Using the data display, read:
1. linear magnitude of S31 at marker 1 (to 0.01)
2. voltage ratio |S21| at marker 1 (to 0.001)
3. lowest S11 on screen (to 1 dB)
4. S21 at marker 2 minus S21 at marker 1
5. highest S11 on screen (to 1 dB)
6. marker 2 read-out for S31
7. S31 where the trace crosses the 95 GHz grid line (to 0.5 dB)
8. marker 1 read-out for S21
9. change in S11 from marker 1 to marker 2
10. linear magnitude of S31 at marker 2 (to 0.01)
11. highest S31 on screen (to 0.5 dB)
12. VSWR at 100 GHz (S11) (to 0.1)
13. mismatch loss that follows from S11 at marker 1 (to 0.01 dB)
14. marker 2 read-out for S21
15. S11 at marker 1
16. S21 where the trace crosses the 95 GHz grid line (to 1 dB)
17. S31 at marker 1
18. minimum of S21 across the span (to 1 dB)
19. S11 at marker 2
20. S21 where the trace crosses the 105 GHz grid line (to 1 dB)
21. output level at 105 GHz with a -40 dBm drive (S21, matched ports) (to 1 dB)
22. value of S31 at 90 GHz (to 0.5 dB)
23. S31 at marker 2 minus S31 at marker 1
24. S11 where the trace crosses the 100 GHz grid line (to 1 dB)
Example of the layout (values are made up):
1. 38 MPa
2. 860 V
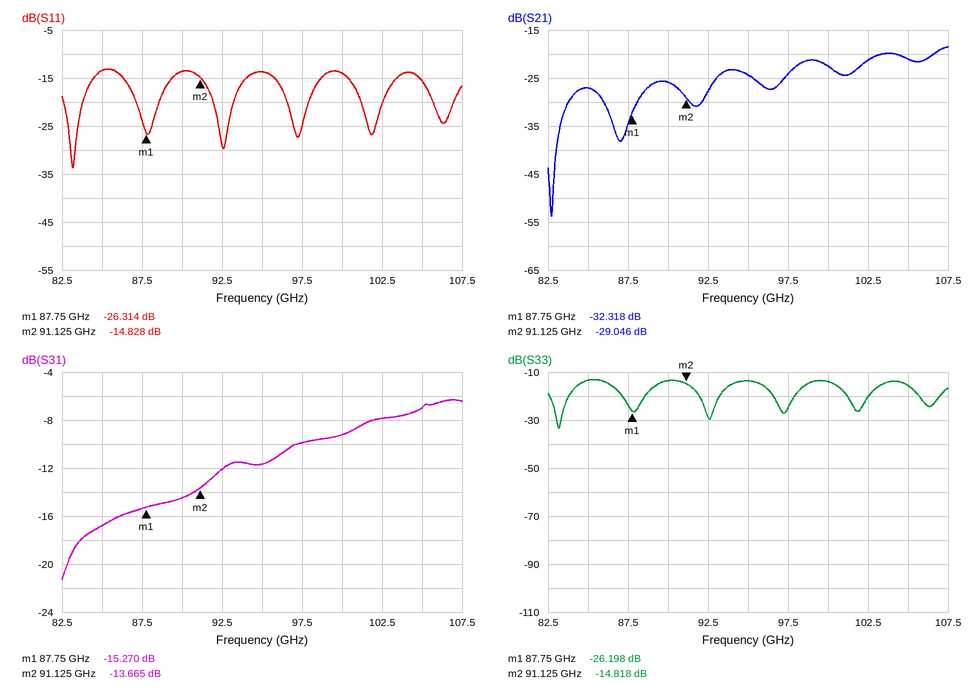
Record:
1. 0.17
2. 0.024
3. -34 dB
4. 3.272 dB
5. -13 dB
6. -13.665 dB
7. -11.5 dB
8. -32.318 dB
9. 11.486 dB
10. 0.21
11. -6.5 dB
12. 1.5
13. 0.01 dB
14. -29.046 dB
15. -26.314 dB
16. -24 dB
17. -15.270 dB
18. -54 dB
19. -14.828 dB
20. -21 dB
21. -61 dBm
22. -14.5 dB
23. 1.605 dB
24. -14 dB
